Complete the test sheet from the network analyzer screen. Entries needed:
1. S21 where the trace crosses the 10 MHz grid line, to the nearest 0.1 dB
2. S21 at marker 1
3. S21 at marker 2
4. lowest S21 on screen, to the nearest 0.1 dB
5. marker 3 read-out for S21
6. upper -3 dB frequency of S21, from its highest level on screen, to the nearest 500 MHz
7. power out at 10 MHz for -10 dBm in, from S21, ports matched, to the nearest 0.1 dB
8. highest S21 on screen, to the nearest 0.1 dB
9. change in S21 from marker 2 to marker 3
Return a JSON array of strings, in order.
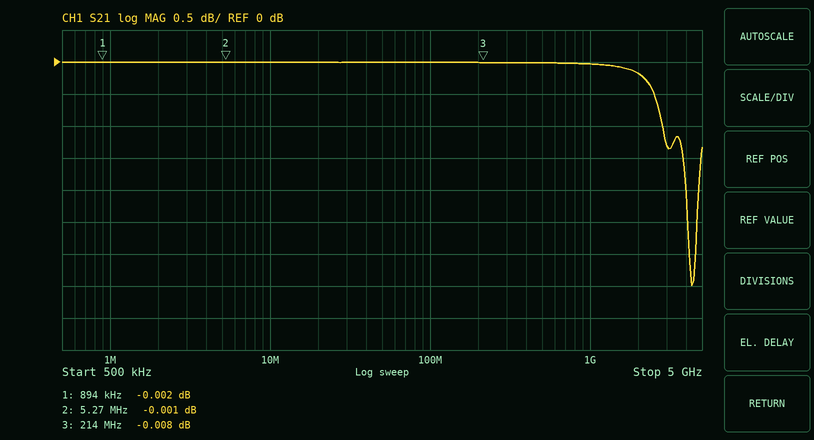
["0.0 dB", "-0.002 dB", "-0.001 dB", "-3.5 dB", "-0.008 dB", "4.0 GHz", "-10.0 dBm", "0.0 dB", "-0.007 dB"]
